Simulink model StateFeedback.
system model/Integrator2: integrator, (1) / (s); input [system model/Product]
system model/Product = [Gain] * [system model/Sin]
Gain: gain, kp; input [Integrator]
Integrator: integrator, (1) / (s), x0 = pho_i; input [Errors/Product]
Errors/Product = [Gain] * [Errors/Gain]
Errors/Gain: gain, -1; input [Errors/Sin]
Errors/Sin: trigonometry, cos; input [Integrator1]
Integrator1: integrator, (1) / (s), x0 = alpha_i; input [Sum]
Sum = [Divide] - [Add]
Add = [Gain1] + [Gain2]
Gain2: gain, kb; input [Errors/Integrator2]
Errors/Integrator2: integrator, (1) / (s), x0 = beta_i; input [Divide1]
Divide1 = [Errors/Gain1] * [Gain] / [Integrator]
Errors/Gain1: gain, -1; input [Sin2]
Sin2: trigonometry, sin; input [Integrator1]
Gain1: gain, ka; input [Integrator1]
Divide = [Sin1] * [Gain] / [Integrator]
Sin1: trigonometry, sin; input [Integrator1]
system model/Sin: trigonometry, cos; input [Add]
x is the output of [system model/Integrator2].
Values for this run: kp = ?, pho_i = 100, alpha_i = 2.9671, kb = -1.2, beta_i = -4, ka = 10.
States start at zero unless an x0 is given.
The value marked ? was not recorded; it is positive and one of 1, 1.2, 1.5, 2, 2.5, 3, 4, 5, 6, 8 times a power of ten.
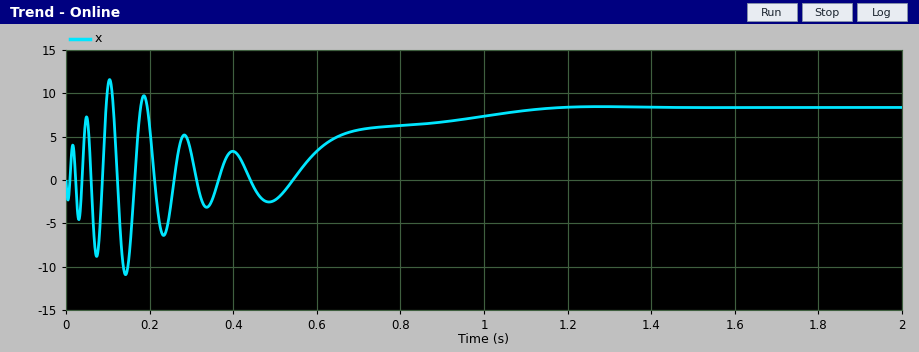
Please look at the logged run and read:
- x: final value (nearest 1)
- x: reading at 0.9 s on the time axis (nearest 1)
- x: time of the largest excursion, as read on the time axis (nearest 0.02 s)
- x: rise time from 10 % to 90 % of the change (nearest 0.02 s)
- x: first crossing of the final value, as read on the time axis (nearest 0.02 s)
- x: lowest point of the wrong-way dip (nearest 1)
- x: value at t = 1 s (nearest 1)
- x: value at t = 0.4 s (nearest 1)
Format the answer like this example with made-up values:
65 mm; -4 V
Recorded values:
8; 7; 0.10 s; 0.08 s; 0.10 s; -11; 7; 3
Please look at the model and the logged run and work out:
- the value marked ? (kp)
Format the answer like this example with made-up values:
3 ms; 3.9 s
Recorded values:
8
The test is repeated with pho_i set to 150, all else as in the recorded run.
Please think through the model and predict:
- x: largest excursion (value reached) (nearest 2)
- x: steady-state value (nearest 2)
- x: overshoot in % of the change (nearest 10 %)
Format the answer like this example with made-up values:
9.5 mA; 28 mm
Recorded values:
18; 12; 40 %
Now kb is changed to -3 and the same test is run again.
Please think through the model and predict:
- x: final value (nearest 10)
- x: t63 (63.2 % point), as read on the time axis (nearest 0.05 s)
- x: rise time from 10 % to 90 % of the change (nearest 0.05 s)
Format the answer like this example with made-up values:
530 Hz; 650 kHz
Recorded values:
-100; 0.65 s; 0.30 s
